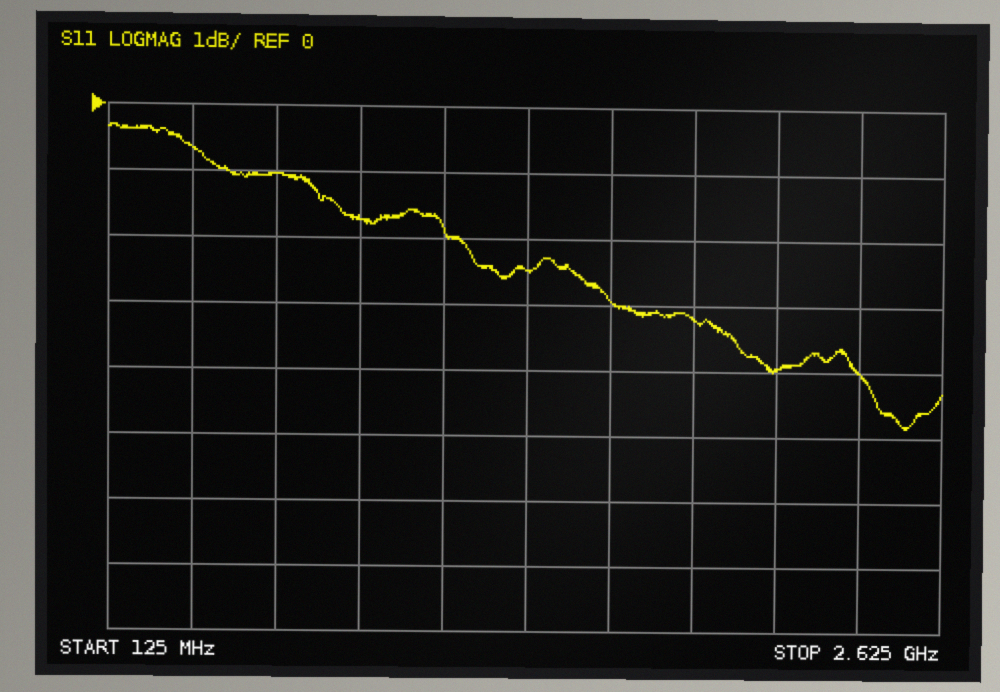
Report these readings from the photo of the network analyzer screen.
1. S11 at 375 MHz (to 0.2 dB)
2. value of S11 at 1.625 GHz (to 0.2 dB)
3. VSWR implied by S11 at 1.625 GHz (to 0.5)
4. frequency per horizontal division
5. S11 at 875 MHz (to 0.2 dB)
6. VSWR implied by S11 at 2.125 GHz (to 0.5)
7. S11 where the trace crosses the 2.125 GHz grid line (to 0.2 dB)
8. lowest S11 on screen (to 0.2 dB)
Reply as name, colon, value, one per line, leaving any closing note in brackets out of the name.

S11 at 375 MHz: -0.6 dB
value of S11 at 1.625 GHz: -3.0 dB
VSWR implied by S11 at 1.625 GHz: 6.0
frequency per horizontal division: 250 MHz
S11 at 875 MHz: -1.8 dB
VSWR implied by S11 at 2.125 GHz: 4.5
S11 where the trace crosses the 2.125 GHz grid line: -4.0 dB
lowest S11 on screen: -4.8 dB
